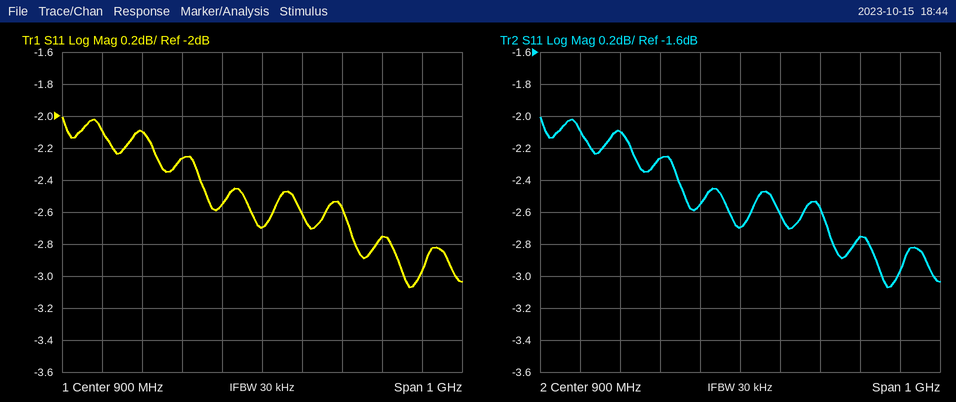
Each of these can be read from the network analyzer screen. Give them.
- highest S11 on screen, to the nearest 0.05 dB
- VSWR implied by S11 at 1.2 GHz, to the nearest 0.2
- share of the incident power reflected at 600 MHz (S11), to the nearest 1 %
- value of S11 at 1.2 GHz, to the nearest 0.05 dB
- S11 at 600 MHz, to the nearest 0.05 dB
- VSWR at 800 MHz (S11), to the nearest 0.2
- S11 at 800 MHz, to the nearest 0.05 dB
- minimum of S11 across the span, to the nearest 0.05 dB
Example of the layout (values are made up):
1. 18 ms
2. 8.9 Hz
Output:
1. -2.00 dB
2. 6.4
3. 62 %
4. -2.75 dB
5. -2.10 dB
6. 6.8
7. -2.55 dB
8. -3.05 dB
